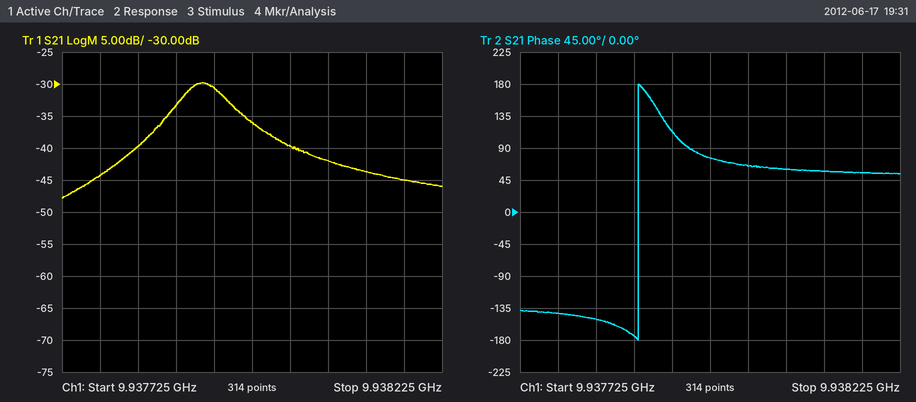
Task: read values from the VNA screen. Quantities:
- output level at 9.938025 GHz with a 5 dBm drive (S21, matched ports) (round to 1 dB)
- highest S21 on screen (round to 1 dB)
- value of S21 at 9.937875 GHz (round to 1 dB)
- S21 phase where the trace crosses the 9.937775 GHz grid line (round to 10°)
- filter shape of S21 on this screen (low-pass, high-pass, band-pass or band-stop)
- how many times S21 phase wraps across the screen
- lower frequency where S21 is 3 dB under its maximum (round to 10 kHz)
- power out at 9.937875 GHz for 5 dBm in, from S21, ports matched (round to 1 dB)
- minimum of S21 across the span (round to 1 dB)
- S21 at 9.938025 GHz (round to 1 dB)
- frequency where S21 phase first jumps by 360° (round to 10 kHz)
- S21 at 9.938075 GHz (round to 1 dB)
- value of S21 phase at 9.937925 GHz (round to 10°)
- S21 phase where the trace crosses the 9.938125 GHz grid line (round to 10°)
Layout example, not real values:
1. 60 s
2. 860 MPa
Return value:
1. -35 dBm
2. -30 dB
3. -33 dB
4. -140°
5. band-pass
6. 1
7. 9.93788 GHz
8. -28 dBm
9. -48 dB
10. -40 dB
11. 9.93788 GHz
12. -42 dB
13. 110°
14. 60°
